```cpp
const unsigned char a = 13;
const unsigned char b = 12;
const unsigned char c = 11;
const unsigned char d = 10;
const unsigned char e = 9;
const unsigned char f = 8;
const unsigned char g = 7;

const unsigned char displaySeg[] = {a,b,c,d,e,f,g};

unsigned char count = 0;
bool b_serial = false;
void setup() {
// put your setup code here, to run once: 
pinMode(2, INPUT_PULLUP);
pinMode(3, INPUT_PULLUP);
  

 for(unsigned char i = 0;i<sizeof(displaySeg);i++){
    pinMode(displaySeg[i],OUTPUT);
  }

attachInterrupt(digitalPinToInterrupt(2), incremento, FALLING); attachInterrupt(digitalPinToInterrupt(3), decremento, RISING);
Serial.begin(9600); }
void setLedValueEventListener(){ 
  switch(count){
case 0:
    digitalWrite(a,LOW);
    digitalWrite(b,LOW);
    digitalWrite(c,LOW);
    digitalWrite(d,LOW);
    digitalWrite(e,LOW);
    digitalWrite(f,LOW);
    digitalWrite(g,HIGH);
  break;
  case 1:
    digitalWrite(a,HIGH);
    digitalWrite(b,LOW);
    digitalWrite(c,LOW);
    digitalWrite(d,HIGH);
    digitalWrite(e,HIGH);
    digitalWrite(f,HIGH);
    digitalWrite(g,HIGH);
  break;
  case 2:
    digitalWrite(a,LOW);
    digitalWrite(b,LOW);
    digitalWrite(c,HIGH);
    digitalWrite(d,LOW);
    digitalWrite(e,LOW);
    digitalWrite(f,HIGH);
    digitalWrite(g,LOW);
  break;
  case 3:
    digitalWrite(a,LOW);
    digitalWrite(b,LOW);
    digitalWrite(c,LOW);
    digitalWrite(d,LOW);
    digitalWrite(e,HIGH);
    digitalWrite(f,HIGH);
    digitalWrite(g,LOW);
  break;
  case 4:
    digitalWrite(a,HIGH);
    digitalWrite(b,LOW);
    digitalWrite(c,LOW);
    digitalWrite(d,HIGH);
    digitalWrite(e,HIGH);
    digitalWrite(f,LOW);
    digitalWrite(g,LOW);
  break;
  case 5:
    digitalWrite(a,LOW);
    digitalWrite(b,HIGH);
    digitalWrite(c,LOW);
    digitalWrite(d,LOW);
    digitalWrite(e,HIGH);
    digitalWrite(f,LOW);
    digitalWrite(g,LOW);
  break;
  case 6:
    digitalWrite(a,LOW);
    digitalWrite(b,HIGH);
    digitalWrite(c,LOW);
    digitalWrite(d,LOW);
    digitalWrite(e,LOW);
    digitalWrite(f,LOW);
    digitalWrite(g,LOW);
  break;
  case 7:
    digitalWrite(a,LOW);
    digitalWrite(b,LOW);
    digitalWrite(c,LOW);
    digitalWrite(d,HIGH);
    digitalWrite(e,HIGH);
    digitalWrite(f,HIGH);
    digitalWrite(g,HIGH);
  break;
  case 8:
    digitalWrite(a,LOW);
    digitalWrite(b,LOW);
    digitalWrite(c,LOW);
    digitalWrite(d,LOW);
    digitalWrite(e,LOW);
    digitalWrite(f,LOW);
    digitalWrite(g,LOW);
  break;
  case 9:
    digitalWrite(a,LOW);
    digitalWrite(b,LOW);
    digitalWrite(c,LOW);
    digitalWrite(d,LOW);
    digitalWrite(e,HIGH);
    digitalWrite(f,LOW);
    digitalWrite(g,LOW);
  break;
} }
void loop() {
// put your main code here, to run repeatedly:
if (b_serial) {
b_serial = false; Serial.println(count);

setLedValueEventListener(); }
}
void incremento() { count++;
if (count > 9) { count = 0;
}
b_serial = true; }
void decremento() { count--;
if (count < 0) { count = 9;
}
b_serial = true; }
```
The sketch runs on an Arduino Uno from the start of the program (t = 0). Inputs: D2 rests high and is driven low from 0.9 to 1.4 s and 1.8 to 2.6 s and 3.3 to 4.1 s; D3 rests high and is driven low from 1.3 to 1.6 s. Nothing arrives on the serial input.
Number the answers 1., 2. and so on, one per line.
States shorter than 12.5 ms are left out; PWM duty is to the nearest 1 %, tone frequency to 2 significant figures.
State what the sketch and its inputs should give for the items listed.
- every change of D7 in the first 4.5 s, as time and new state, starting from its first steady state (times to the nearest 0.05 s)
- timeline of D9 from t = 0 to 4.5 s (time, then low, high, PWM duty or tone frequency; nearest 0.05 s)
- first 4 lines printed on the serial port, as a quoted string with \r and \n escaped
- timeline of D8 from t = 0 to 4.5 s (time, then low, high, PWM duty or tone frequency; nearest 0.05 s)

1. 0 s low; 0.9 s high; 3.3 s low
2. 0 s low; 0.9 s high; 1.6 s low; 1.8 s high; 3.3 s low
3. "1\r\n0\r\n1\r\n2\r\n"
4. 0 s low; 0.9 s high; 1.6 s low; 1.8 s high
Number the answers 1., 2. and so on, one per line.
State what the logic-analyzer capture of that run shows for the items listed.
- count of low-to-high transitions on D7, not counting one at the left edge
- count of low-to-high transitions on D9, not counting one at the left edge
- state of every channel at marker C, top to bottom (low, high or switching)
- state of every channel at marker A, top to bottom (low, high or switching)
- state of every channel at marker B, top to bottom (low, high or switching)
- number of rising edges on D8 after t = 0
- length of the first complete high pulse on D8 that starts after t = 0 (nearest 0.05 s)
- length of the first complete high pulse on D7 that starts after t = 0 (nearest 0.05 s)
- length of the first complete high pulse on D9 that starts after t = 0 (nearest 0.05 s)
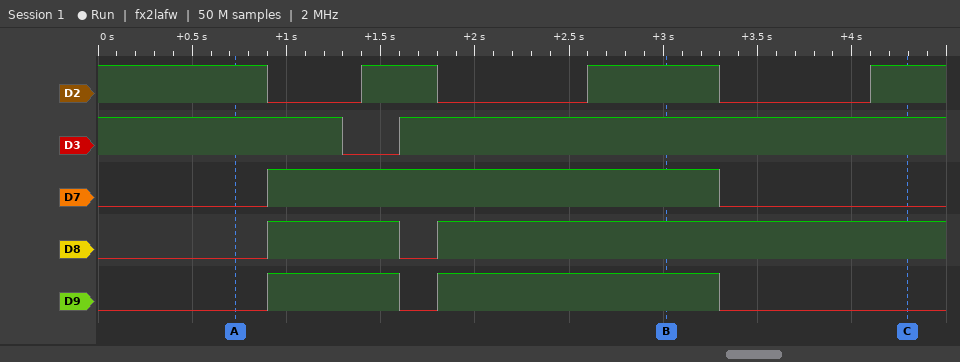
1. 1
2. 2
3. D2 high, D3 high, D7 low, D8 high, D9 low
4. D2 high, D3 high, D7 low, D8 low, D9 low
5. D2 high, D3 high, D7 high, D8 high, D9 high
6. 2
7. 0.70 s
8. 2.40 s
9. 0.70 s
